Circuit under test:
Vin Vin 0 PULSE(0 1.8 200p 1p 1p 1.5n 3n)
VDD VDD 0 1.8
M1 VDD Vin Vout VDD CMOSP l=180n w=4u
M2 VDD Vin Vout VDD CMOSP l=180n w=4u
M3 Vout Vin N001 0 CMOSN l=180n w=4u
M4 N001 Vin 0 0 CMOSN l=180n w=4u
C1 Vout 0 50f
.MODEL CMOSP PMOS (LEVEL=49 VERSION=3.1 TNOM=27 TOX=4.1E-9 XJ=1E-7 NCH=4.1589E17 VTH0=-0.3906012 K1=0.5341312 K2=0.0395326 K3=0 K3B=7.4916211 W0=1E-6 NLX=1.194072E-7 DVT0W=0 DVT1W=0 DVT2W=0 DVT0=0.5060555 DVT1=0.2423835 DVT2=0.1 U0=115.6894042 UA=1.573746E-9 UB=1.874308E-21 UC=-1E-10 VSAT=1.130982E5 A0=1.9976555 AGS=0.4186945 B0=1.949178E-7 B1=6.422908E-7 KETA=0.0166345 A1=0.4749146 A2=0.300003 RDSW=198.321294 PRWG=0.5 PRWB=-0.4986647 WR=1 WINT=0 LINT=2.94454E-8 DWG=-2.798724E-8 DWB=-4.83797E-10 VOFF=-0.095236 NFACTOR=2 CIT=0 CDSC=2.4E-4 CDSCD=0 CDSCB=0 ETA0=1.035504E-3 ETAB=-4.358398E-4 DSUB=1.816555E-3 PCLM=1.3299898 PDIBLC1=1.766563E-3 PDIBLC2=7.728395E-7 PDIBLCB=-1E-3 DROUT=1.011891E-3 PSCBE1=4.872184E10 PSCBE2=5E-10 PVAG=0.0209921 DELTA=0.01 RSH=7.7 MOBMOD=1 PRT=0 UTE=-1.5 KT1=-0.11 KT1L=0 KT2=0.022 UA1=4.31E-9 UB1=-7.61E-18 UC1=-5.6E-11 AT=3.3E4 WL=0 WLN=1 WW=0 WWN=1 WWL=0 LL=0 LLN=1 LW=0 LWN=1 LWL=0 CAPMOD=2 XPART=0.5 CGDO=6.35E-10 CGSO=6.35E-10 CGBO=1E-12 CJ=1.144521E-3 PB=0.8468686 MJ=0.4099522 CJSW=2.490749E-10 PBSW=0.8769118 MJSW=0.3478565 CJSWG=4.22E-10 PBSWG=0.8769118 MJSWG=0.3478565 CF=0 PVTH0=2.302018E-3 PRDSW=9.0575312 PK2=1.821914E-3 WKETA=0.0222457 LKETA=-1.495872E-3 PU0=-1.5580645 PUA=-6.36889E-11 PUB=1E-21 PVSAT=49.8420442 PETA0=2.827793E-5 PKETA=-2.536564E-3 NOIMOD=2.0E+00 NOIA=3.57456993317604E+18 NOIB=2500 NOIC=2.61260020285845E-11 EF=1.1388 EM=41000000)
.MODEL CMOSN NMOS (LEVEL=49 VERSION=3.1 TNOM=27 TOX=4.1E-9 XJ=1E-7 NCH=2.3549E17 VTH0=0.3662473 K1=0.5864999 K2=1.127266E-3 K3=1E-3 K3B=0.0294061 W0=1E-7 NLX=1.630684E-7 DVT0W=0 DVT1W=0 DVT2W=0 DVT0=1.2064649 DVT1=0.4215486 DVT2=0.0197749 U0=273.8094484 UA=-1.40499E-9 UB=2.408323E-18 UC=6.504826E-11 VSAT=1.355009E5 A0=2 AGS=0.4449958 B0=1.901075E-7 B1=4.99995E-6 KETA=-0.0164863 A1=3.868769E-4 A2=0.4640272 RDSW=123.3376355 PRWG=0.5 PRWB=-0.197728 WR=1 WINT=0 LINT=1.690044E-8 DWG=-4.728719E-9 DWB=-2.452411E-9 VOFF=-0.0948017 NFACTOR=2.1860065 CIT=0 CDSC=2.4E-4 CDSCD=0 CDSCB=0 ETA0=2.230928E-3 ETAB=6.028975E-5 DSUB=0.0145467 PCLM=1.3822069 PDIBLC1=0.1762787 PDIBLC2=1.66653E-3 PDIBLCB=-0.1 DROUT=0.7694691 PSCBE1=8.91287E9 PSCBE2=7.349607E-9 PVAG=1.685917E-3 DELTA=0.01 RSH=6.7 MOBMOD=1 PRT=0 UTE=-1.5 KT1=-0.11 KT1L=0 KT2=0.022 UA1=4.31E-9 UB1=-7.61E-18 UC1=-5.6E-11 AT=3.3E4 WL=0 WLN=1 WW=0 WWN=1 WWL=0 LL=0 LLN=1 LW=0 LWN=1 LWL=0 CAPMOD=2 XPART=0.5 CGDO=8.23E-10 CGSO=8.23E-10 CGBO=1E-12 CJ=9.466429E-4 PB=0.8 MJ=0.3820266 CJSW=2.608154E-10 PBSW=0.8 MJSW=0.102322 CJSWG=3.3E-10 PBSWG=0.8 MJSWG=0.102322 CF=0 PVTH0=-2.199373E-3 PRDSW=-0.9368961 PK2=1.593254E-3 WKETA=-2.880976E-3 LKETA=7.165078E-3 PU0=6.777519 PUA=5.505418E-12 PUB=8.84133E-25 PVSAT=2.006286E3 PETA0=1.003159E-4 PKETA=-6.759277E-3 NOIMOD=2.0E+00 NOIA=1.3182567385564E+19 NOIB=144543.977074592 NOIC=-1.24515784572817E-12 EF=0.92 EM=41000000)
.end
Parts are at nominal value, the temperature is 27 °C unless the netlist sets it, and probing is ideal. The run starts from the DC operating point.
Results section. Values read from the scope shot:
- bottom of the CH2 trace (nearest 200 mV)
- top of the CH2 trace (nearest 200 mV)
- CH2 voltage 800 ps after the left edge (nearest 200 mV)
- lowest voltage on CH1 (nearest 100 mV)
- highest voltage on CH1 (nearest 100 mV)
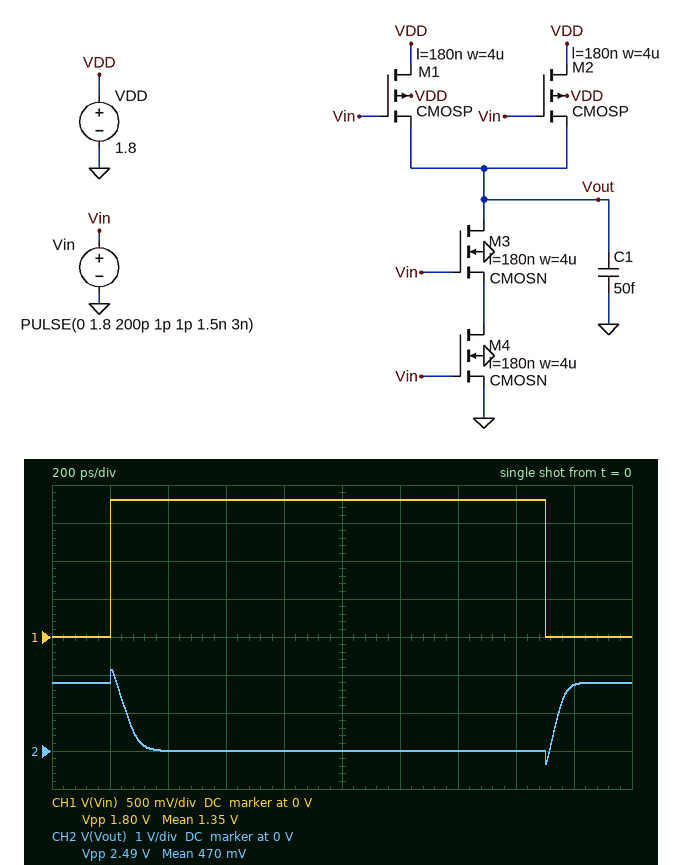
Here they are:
-400 mV
2.2 V
0 V
0 V
1.8 V
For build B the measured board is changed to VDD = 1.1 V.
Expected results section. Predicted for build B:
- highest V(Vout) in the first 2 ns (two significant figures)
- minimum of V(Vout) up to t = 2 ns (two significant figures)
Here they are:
1.4 V
-370 mV
